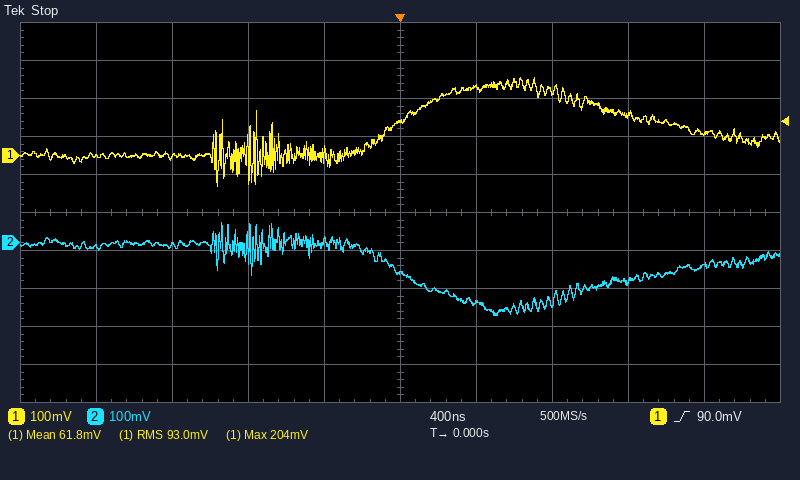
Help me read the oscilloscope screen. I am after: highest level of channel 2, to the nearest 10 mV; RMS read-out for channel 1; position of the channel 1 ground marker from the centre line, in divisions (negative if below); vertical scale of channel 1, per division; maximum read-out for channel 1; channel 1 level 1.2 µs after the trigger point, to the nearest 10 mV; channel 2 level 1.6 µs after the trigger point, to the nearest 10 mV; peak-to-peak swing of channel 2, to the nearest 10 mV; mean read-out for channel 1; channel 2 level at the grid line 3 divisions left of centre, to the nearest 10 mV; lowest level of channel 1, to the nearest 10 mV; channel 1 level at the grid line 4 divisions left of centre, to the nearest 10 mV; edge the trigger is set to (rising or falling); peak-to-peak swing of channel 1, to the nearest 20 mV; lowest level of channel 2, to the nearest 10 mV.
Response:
50 mV
93.0 mV
+1.5 div
100 mV
204 mV
110 mV
-60 mV
240 mV
61.8 mV
-10 mV
-80 mV
0 mV
rising
280 mV
-190 mV
